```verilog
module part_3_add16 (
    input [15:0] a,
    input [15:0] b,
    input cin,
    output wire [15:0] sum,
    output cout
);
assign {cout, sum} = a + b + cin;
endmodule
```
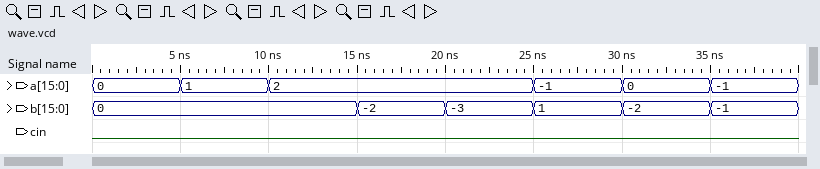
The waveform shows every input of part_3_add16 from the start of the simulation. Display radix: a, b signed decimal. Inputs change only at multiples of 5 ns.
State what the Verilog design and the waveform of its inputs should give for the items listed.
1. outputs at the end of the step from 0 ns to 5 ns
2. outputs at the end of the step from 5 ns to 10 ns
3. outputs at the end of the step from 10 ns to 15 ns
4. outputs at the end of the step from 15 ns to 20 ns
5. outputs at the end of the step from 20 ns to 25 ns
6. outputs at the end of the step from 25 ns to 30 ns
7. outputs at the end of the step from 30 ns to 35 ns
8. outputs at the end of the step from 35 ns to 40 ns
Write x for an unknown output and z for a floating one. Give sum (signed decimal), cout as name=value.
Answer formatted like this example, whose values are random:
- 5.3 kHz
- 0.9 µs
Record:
- sum=0, cout=0
- sum=1, cout=0
- sum=2, cout=0
- sum=0, cout=1
- sum=-1, cout=0
- sum=0, cout=1
- sum=-2, cout=0
- sum=-2, cout=1
